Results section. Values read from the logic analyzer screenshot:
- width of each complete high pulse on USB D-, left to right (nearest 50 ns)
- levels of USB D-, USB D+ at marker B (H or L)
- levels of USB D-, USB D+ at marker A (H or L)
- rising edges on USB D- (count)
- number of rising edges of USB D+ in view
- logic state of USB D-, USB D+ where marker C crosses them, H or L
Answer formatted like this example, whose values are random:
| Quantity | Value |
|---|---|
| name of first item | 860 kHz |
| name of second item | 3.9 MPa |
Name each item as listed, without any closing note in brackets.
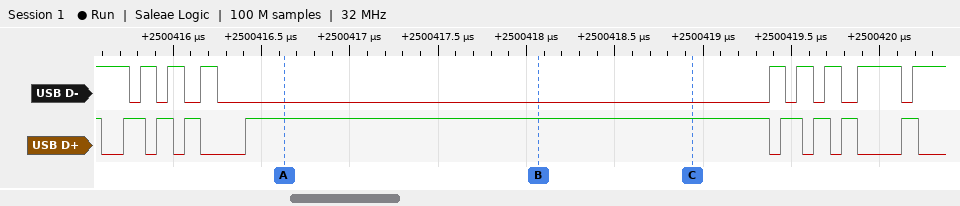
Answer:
| Quantity | Value |
|---|---|
| width of each complete high pulse on USB D-, left to right | 100 ns, 100 ns, 100 ns, 100 ns, 100 ns, 100 ns, 250 ns |
| levels of USB D-, USB D+ at marker B | USB D-=L, USB D+=H |
| levels of USB D-, USB D+ at marker A | USB D-=L, USB D+=H |
| rising edges on USB D- | 8 |
| number of rising edges of USB D+ in view | 8 |
| logic state of USB D-, USB D+ where marker C crosses them, H or L | USB D-=L, USB D+=H |
